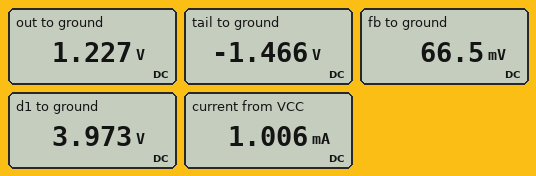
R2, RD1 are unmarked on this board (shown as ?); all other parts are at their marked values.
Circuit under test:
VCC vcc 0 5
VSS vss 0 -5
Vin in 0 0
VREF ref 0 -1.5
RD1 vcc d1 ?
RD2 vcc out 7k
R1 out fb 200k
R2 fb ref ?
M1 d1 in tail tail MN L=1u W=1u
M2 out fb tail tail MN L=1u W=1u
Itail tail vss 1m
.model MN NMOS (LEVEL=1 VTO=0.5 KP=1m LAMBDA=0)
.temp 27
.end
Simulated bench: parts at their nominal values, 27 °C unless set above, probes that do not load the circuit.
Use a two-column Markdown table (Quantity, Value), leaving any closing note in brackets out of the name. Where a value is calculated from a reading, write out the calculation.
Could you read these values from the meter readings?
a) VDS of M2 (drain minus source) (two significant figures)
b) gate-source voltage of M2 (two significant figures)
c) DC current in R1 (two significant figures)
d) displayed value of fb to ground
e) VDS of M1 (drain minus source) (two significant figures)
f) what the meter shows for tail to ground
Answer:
| Quantity | Value |
|---|---|
| VDS of M2 (drain minus source) | 1.227 V - (-1.466 V) = 2.7 V |
| gate-source voltage of M2 | 66.5 mV - (-1.466 V) = 1.5 V |
| DC current in R1 | (1.227 V - 66.5 mV) / 200 kΩ = 5.8 µA |
| displayed value of fb to ground | 66.5 mV |
| VDS of M1 (drain minus source) | 3.973 V - (-1.466 V) = 5.4 V |
| what the meter shows for tail to ground | -1.466 V |
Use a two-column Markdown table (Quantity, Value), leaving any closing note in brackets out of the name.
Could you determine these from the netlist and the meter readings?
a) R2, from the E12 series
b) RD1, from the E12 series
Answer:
| Quantity | Value |
|---|---|
| R2, from the E12 series | 270 kΩ |
| RD1, from the E12 series | 2.2 kΩ |
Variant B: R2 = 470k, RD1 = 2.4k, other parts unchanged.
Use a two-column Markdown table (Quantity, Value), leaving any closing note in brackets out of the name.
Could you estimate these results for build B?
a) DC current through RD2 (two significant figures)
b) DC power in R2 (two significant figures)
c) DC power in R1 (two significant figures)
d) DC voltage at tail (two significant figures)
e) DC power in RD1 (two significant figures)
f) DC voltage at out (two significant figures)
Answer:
| Quantity | Value |
|---|---|
| DC current through RD2 | 590 µA |
| DC power in R2 | 5.9 µW |
| DC power in R1 | 2.5 µW |
| DC voltage at tail | -1.4 V |
| DC power in RD1 | 410 µW |
| DC voltage at out | 880 mV |
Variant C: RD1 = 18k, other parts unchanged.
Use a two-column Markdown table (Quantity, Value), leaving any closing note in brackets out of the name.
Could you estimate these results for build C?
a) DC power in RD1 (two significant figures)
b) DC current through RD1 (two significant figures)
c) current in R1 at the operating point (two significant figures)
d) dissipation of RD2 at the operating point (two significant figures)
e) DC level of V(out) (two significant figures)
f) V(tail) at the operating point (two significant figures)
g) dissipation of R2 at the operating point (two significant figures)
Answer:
| Quantity | Value |
|---|---|
| DC power in RD1 | 2.5 mW |
| DC current through RD1 | 370 µA |
| current in R1 at the operating point | 4.4 µA |
| dissipation of RD2 at the operating point | 2.8 mW |
| DC level of V(out) | 560 mV |
| V(tail) at the operating point | -1.9 V |
| dissipation of R2 at the operating point | 5.2 µW |
